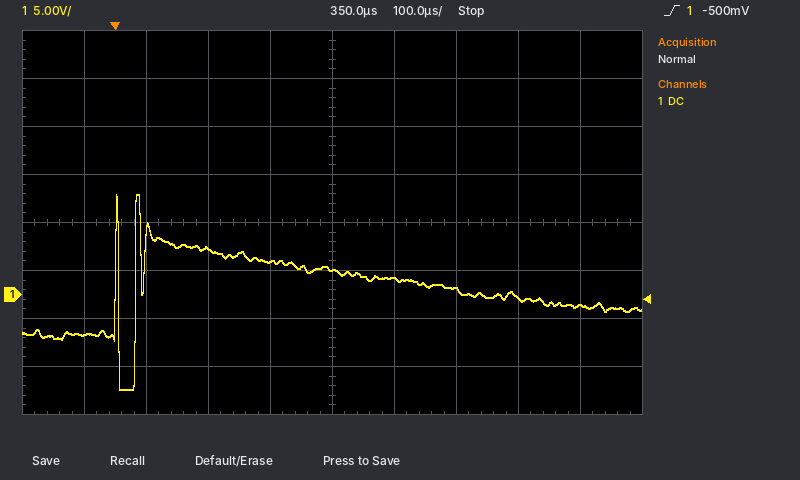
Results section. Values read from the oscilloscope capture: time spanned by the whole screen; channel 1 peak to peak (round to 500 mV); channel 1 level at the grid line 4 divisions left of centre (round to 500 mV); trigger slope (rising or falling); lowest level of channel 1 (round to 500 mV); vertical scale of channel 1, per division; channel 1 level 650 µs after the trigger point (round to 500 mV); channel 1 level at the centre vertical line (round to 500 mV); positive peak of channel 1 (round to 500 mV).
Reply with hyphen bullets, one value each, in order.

- 1 ms
- 20.5 V
- -4.0 V
- rising
- -10.0 V
- 5 V
- -500 mV
- 2.5 V
- 10.5 V
